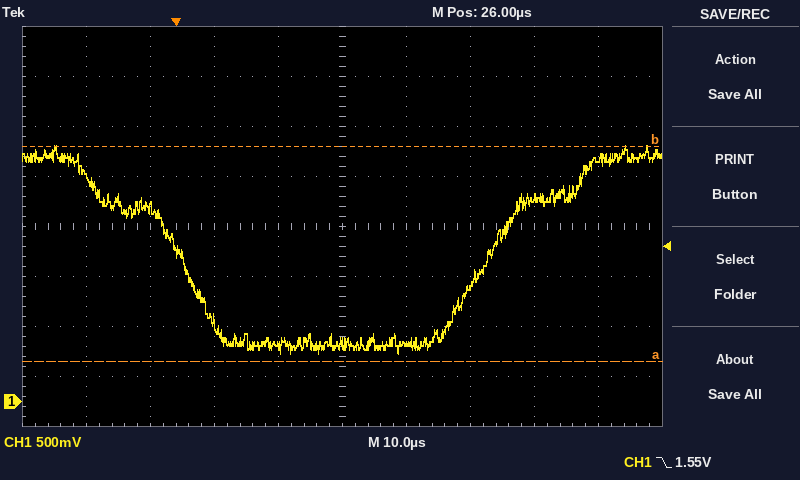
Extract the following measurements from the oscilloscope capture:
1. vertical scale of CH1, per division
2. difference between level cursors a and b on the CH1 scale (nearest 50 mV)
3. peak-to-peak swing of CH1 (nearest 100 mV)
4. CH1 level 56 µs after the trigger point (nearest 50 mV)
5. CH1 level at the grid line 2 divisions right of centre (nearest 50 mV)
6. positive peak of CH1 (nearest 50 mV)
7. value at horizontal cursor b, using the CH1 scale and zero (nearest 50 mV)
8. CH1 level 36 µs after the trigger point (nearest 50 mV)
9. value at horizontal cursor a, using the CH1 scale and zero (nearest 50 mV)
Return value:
500 mV
2.15 V
2.10 V
2.05 V
1.15 V
2.55 V
2.55 V
600 mV
400 mV
